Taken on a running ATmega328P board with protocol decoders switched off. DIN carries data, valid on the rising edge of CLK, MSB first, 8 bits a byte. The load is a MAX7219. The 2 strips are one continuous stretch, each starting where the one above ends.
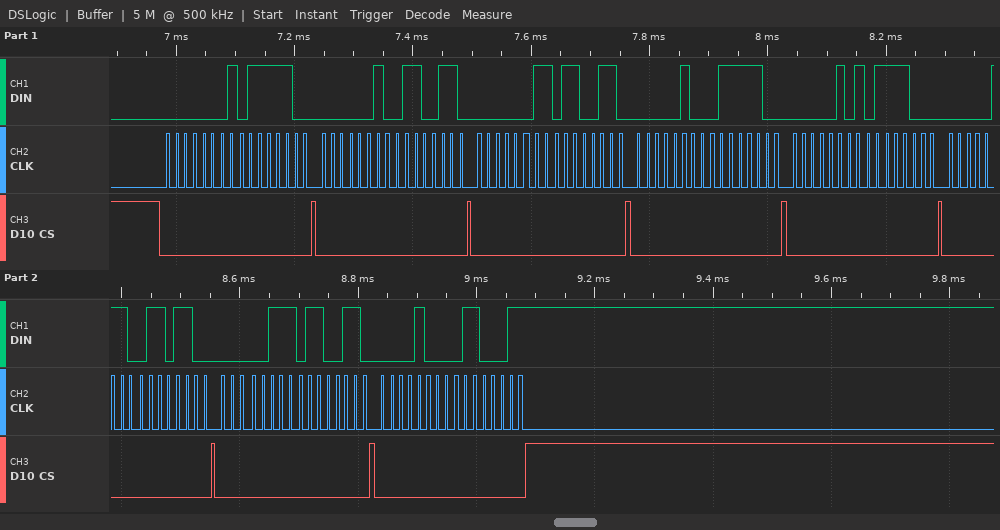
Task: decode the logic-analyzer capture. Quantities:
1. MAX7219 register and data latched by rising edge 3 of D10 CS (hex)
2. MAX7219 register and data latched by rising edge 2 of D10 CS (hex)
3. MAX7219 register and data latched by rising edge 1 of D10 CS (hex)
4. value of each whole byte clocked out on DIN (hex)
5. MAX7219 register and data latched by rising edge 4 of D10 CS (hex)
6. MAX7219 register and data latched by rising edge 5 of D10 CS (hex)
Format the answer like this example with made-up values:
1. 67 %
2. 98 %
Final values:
1. register 0x3, data 0x66
2. register 0x2, data 0x66
3. register 0x1, data 0x7C
4. 01 7C 02 66 03 66 04 7C 05 78 06 6C 07 66 08 63
5. register 0x4, data 0x7C
6. register 0x5, data 0x78
